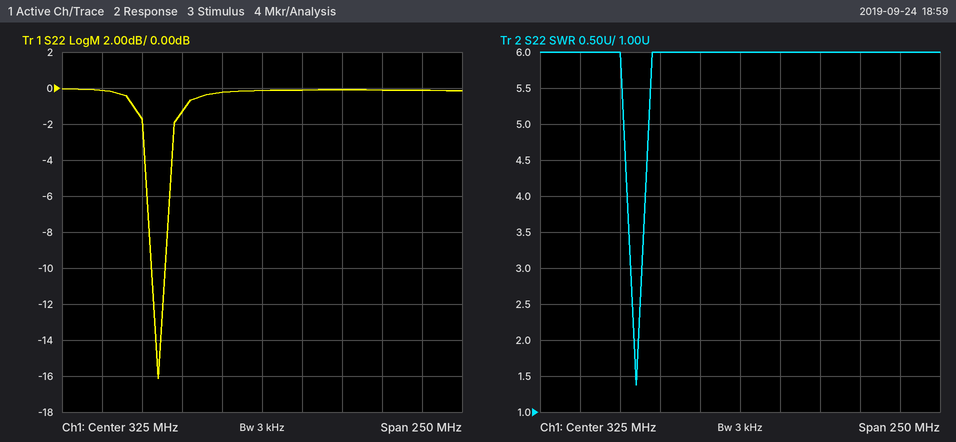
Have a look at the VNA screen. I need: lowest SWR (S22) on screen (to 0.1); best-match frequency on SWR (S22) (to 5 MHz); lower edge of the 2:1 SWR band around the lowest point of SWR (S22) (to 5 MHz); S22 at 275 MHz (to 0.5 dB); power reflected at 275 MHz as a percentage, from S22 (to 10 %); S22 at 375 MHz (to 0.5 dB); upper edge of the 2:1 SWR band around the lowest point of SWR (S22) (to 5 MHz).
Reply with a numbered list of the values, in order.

1. 1.4
2. 260 MHz
3. 260 MHz
4. -1.5 dB
5. 70 %
6. 0.0 dB
7. 260 MHz
